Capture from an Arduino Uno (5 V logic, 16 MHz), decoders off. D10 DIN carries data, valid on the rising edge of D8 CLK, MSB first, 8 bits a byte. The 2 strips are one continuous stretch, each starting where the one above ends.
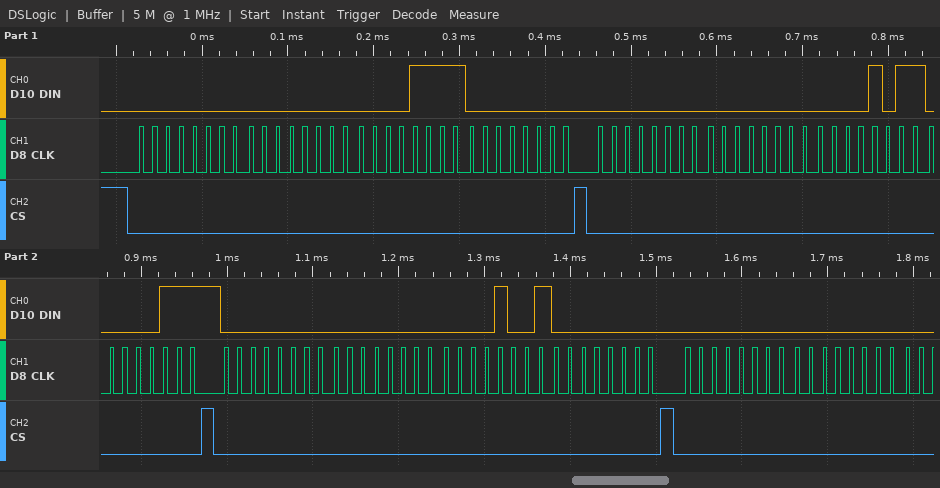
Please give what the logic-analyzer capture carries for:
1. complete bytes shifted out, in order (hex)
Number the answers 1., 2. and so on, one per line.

1. 00 00 0F 00 00 00 0B 07 00 00 09 00 00 00
